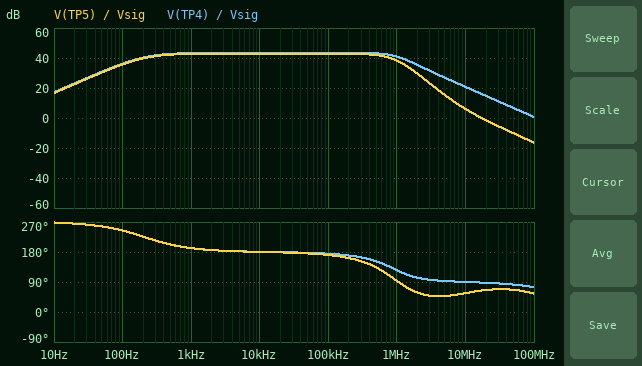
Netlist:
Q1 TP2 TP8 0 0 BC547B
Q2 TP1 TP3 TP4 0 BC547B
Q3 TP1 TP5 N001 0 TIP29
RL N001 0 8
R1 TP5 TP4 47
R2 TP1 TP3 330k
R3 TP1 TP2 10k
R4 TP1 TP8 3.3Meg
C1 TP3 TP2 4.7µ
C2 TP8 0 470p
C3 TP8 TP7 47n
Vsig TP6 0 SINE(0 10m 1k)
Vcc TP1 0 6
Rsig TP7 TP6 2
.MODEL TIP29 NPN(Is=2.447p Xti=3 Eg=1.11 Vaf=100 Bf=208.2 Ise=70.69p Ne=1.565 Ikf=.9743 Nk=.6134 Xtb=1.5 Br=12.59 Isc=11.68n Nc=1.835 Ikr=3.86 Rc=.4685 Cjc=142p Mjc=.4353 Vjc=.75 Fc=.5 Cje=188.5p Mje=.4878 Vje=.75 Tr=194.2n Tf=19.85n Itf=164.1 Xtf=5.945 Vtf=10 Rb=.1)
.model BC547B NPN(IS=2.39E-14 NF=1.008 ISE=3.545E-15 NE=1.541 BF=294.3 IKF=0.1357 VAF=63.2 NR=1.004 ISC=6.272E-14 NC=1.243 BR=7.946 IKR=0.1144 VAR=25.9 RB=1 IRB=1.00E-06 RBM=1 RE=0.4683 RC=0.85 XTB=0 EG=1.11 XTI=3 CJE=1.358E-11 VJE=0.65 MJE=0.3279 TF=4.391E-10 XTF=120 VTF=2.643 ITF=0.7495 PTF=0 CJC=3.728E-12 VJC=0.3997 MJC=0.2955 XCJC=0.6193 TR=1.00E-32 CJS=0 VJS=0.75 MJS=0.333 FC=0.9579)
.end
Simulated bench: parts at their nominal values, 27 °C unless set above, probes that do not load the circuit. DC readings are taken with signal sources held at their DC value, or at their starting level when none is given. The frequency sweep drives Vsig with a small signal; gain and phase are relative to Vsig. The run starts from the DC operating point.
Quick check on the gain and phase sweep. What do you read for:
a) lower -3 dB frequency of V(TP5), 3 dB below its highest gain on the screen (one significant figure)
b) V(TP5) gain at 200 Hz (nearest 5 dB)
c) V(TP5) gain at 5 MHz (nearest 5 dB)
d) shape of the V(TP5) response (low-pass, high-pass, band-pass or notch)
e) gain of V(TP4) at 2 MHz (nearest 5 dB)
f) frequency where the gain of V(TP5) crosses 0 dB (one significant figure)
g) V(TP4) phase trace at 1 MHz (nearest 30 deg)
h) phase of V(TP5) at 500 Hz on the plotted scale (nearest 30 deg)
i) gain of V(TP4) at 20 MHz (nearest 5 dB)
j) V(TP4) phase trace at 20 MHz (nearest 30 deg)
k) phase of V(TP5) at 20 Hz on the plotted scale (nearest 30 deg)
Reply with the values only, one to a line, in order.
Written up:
200 Hz
40 dB
15 dB
band-pass
35 dB
20 MHz
120 deg
210 deg
15 dB
90 deg
270 deg
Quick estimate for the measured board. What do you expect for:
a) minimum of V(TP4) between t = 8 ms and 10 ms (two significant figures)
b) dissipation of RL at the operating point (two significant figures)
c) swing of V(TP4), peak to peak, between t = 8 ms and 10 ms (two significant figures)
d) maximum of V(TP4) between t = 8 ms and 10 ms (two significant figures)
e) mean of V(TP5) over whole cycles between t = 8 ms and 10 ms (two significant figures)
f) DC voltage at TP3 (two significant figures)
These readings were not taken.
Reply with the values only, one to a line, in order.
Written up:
1.5 V
470 mW
2.6 V
4.1 V
2.8 V
3.4 V
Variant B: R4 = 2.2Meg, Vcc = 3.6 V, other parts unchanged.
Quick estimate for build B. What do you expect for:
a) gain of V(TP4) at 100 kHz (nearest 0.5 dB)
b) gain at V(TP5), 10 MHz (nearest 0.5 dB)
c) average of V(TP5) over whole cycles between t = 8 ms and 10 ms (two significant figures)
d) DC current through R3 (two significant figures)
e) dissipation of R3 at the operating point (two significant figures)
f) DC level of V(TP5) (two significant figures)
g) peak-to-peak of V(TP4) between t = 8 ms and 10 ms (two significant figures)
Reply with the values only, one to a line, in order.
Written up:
38.5 dB
-4.0 dB
2.1 V
340 µA
1.2 mW
1.6 V
1.4 V
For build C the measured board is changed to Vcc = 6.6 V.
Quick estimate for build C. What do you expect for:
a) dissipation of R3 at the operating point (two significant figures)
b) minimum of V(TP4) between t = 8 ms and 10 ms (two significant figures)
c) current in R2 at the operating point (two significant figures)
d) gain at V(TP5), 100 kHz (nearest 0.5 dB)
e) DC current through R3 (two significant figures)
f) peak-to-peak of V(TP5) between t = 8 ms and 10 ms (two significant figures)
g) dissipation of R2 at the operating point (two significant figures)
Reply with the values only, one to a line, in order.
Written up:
2.7 mW
1.7 V
9.0 µA
43.5 dB
520 µA
2.7 V
27 µW
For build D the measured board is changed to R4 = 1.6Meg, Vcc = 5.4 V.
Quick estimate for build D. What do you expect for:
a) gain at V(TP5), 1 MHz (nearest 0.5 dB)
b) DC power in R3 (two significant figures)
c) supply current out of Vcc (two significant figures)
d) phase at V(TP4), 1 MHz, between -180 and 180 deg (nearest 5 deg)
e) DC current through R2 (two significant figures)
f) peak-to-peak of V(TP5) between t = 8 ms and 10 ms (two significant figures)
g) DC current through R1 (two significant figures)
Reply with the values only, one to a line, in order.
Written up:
29.0 dB
2.8 mW
210 mA
135 deg
7.0 µA
1.1 V
2.0 mA
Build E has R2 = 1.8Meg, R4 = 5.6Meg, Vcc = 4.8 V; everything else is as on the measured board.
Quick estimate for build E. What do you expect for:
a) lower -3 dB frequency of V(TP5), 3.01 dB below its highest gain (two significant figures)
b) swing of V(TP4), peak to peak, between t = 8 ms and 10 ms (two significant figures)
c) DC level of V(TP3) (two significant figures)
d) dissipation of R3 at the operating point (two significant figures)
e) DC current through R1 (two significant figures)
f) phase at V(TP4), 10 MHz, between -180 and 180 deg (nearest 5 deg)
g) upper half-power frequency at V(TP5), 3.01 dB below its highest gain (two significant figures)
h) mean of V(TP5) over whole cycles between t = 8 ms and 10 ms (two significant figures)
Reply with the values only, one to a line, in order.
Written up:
96 Hz
1.3 V
1.7 V
480 µW
520 µA
90 deg
640 kHz
1.0 V
